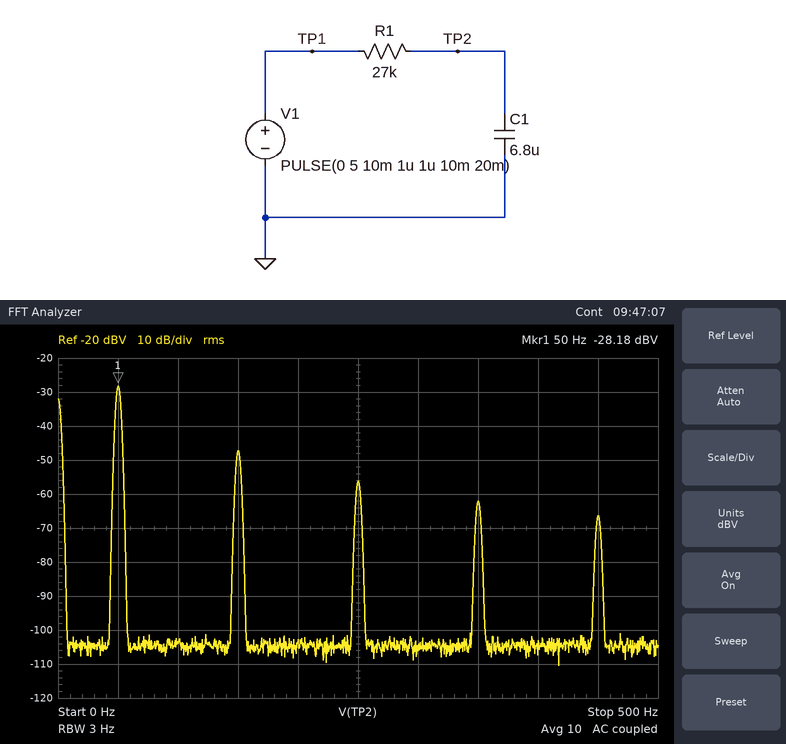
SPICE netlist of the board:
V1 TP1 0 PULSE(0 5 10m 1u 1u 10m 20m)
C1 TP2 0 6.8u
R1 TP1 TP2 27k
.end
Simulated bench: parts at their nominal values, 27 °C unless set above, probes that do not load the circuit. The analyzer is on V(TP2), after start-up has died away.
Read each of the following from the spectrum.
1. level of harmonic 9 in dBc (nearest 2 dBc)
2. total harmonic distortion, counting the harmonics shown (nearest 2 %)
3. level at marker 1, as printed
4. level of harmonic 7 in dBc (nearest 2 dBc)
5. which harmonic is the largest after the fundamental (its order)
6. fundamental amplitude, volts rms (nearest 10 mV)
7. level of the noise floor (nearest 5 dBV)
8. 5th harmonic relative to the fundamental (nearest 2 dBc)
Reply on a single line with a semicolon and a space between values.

-38 dBc; 12 %; -28.18 dBV; -34 dBc; 3; 40 mV; -105 dBV; -28 dBc
